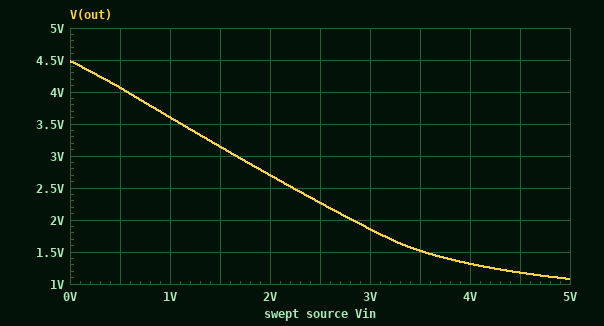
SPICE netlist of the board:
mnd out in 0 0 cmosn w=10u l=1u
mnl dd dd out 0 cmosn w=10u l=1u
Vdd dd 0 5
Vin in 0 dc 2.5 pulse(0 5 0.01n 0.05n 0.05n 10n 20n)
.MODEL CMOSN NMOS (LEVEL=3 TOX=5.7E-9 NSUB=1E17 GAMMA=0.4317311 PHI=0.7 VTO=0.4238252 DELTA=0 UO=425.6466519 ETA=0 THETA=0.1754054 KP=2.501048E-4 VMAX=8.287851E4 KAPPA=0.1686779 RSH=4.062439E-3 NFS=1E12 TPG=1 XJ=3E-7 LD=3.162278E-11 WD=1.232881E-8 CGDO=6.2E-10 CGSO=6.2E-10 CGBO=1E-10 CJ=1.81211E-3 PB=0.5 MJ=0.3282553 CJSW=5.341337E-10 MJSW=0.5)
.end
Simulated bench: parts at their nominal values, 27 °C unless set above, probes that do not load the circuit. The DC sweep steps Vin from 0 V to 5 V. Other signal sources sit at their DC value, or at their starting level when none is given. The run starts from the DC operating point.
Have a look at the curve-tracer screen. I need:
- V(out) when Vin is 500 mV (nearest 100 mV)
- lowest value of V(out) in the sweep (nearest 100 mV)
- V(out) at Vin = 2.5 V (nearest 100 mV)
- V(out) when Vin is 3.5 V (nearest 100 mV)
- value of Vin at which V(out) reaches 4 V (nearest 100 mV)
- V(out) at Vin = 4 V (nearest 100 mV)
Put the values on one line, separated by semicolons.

4.1 V; 1.1 V; 2.3 V; 1.5 V; 600 mV; 1.3 V
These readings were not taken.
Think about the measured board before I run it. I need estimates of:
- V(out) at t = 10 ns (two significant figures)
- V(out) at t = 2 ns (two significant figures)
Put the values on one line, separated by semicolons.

1.1 V; 1.1 V
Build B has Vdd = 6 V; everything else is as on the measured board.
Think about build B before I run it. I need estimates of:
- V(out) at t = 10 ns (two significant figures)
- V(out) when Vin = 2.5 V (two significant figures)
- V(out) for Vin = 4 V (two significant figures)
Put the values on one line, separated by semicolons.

1.5 V; 3.2 V; 2.0 V
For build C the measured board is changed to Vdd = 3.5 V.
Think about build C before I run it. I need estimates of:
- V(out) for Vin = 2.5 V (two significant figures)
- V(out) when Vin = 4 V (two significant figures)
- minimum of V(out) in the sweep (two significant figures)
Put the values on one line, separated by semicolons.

1.0 V; 660 mV; 570 mV
